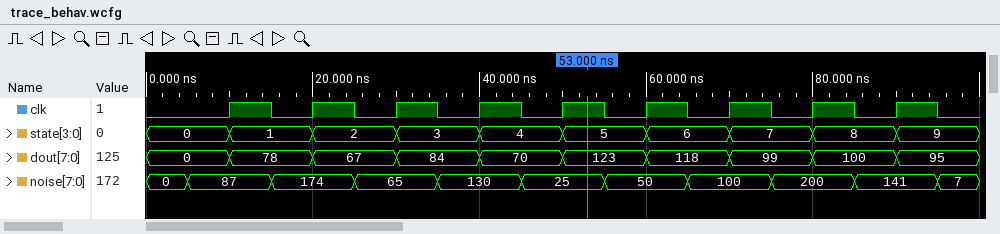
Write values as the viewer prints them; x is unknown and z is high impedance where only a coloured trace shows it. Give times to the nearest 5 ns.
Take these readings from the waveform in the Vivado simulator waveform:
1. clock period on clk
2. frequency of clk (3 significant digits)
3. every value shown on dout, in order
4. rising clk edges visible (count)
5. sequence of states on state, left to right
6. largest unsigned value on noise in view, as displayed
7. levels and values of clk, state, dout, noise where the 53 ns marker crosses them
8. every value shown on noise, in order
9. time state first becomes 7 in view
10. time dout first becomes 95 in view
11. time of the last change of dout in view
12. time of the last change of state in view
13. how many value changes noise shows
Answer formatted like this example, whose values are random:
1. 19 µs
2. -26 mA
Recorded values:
1. 10 ns
2. 100 MHz
3. 0, 78, 67, 84, 70, 123, 118, 99, 100, 95
4. 9
5. 0, 1, 2, 3, 4, 5, 6, 7, 8, 9
6. 200
7. clk=1, state=5, dout=123, noise=25
8. 0, 87, 174, 65, 130, 25, 50, 100, 200, 141, 7
9. 70 ns
10. 90 ns
11. 90 ns
12. 90 ns
13. 10
